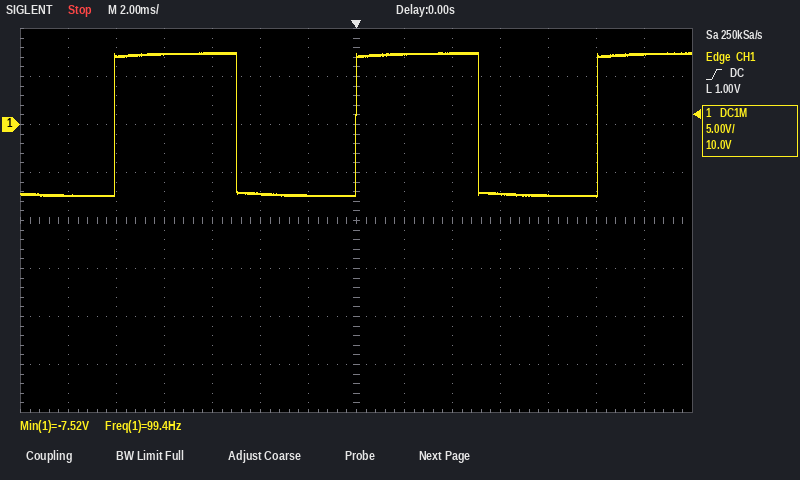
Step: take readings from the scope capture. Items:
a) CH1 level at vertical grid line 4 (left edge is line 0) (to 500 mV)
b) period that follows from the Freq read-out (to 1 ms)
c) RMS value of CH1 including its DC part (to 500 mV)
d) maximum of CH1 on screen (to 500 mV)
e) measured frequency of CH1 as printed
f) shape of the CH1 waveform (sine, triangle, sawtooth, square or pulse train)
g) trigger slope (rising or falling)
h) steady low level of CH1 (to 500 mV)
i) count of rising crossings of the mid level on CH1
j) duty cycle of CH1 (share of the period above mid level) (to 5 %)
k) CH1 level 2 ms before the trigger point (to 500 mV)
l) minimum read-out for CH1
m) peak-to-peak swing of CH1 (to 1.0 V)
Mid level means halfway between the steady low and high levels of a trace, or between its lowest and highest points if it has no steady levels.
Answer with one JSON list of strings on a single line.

["7.5 V", "10 ms", "7.5 V", "7.5 V", "99.4 Hz", "square", "rising", "-7.5 V", "3", "50 %", "-7.5 V", "-7.52 V", "15.0 V"]
